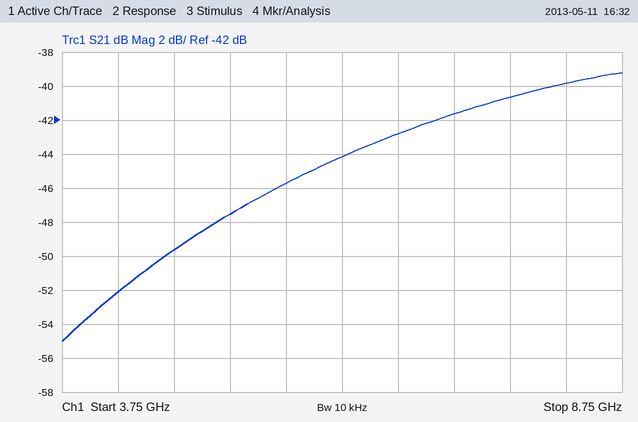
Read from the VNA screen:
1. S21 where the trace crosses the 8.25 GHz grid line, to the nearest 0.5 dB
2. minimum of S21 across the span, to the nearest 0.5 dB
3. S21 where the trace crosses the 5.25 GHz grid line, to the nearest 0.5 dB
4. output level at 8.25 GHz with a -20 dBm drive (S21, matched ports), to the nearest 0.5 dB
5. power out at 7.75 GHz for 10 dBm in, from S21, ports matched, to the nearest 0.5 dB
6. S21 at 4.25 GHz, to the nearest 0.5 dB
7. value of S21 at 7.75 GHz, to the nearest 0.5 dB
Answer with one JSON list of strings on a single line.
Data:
["-40.0 dB", "-55.0 dB", "-47.5 dB", "-60.0 dBm", "-30.5 dBm", "-52.0 dB", "-40.5 dB"]
